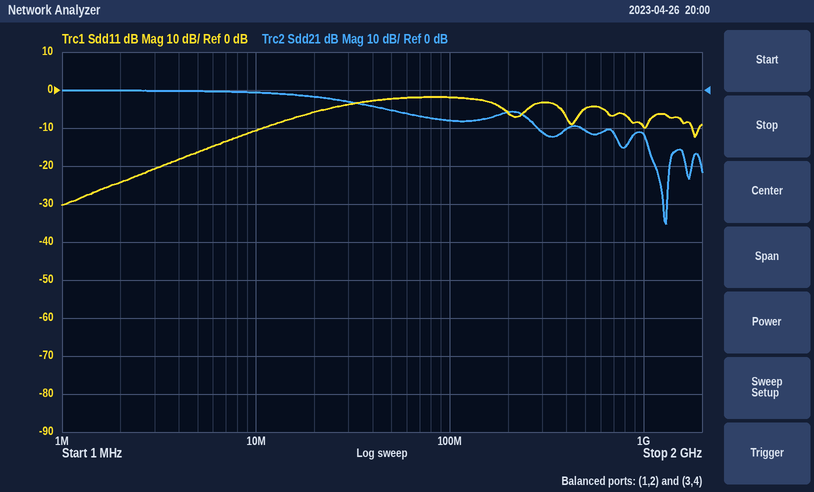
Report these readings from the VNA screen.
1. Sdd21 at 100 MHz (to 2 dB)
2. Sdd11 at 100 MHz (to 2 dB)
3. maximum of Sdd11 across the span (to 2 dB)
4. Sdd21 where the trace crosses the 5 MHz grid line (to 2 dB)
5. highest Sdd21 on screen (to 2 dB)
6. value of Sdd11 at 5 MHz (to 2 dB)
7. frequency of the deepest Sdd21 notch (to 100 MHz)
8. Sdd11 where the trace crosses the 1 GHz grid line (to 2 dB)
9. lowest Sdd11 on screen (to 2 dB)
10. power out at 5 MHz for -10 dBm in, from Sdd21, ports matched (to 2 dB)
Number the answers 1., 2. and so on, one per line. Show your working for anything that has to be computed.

1. -8 dB
2. -2 dB
3. -2 dB
4. 0 dB
5. 0 dB
6. -16 dB
7. 1.3 GHz
8. -10 dB
9. -30 dB
10. -10 dBm + (0 dB) = -10 dBm
